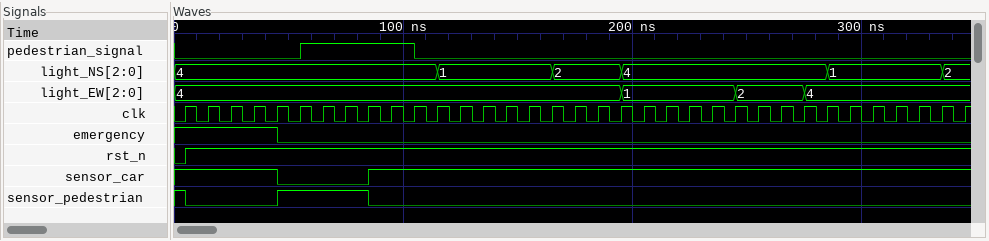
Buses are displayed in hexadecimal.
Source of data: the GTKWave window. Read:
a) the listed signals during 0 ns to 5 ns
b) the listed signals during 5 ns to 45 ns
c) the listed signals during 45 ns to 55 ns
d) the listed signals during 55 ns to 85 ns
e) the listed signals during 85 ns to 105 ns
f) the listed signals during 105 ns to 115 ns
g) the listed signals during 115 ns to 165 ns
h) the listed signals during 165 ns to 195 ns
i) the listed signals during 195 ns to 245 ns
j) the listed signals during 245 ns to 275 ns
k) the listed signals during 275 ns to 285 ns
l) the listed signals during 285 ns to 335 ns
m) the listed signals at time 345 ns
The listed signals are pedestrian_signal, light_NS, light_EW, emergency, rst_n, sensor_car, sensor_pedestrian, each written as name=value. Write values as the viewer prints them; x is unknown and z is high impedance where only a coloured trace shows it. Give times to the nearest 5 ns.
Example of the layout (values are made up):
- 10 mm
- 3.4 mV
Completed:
- pedestrian_signal=0, light_NS=4, light_EW=4, emergency=1, rst_n=0, sensor_car=1, sensor_pedestrian=1
- pedestrian_signal=0, light_NS=4, light_EW=4, emergency=1, rst_n=1, sensor_car=1, sensor_pedestrian=0
- pedestrian_signal=0, light_NS=4, light_EW=4, emergency=0, rst_n=1, sensor_car=0, sensor_pedestrian=1
- pedestrian_signal=1, light_NS=4, light_EW=4, emergency=0, rst_n=1, sensor_car=0, sensor_pedestrian=1
- pedestrian_signal=1, light_NS=4, light_EW=4, emergency=0, rst_n=1, sensor_car=1, sensor_pedestrian=0
- pedestrian_signal=0, light_NS=4, light_EW=4, emergency=0, rst_n=1, sensor_car=1, sensor_pedestrian=0
- pedestrian_signal=0, light_NS=1, light_EW=4, emergency=0, rst_n=1, sensor_car=1, sensor_pedestrian=0
- pedestrian_signal=0, light_NS=2, light_EW=4, emergency=0, rst_n=1, sensor_car=1, sensor_pedestrian=0
- pedestrian_signal=0, light_NS=4, light_EW=1, emergency=0, rst_n=1, sensor_car=1, sensor_pedestrian=0
- pedestrian_signal=0, light_NS=4, light_EW=2, emergency=0, rst_n=1, sensor_car=1, sensor_pedestrian=0
- pedestrian_signal=0, light_NS=4, light_EW=4, emergency=0, rst_n=1, sensor_car=1, sensor_pedestrian=0
- pedestrian_signal=0, light_NS=1, light_EW=4, emergency=0, rst_n=1, sensor_car=1, sensor_pedestrian=0
- pedestrian_signal=0, light_NS=2, light_EW=4, emergency=0, rst_n=1, sensor_car=1, sensor_pedestrian=0
